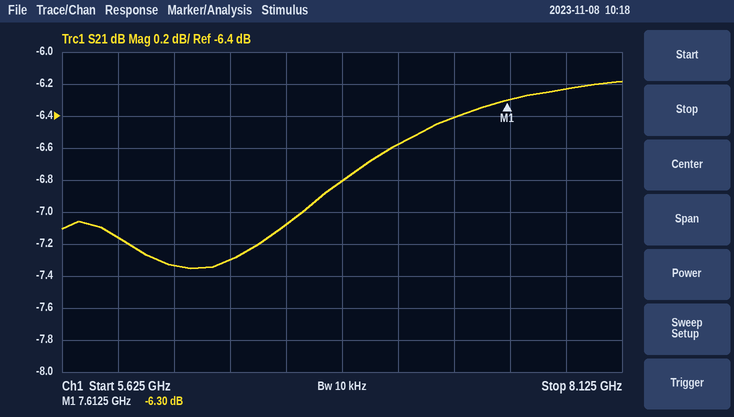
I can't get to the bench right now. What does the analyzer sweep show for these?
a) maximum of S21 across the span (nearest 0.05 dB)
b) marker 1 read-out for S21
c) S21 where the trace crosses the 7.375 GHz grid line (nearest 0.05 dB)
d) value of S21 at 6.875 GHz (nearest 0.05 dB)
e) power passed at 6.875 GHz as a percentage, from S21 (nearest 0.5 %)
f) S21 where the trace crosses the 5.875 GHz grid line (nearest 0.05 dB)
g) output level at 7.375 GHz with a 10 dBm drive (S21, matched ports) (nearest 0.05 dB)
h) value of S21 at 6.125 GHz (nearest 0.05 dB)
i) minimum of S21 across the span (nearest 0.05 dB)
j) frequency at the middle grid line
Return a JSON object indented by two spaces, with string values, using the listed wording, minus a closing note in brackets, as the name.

{
  "maximum of S21 across the span": "-6.20 dB",
  "marker 1 read-out for S21": "-6.30 dB",
  "S21 where the trace crosses the 7.375 GHz grid line": "-6.40 dB",
  "value of S21 at 6.875 GHz": "-6.80 dB",
  "power passed at 6.875 GHz as a percentage, from S21": "21.0 %",
  "S21 where the trace crosses the 5.875 GHz grid line": "-7.15 dB",
  "output level at 7.375 GHz with a 10 dBm drive (S21, matched ports)": "3.60 dBm",
  "value of S21 at 6.125 GHz": "-7.35 dB",
  "minimum of S21 across the span": "-7.35 dB",
  "frequency at the middle grid line": "6.875 GHz"
}
